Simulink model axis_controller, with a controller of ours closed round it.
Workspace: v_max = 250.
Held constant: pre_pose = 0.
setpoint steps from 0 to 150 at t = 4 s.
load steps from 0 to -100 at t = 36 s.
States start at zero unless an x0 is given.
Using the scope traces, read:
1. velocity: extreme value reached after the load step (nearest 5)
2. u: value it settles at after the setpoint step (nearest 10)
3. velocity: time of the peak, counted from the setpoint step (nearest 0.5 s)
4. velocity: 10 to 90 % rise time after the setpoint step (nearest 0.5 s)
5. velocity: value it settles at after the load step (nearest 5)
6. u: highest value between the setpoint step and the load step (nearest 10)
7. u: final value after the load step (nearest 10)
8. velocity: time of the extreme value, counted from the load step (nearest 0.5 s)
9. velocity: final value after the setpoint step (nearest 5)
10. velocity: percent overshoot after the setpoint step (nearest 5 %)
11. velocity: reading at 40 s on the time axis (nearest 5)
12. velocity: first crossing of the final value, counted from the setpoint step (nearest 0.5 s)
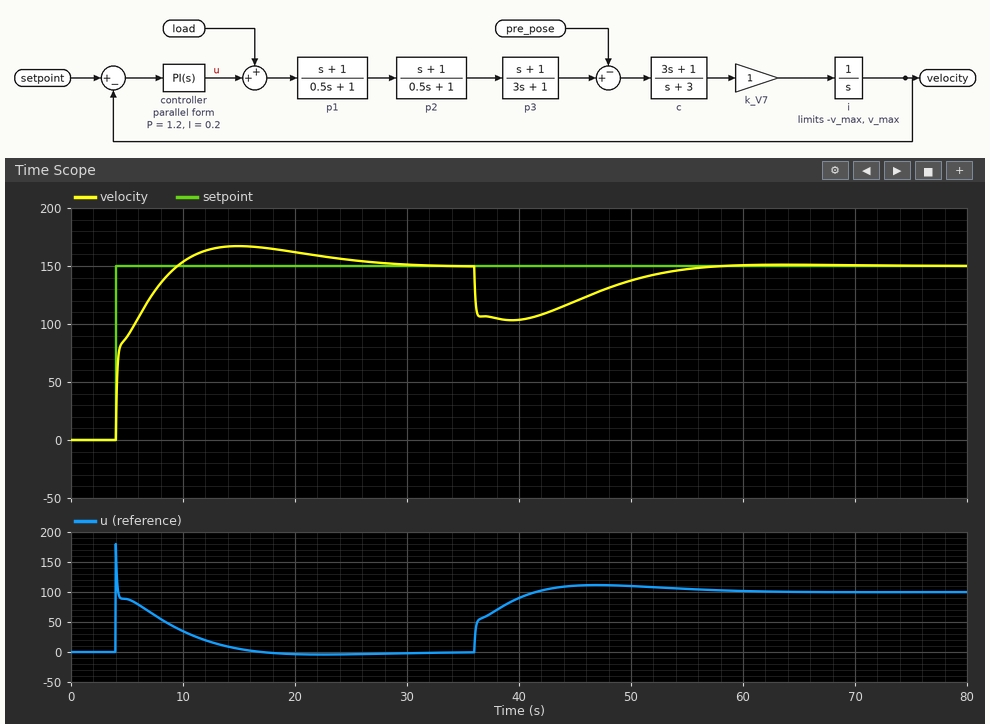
105
0
11.0 s
4.0 s
150
180
100
3.5 s
150
10 %
105
5.5 s
